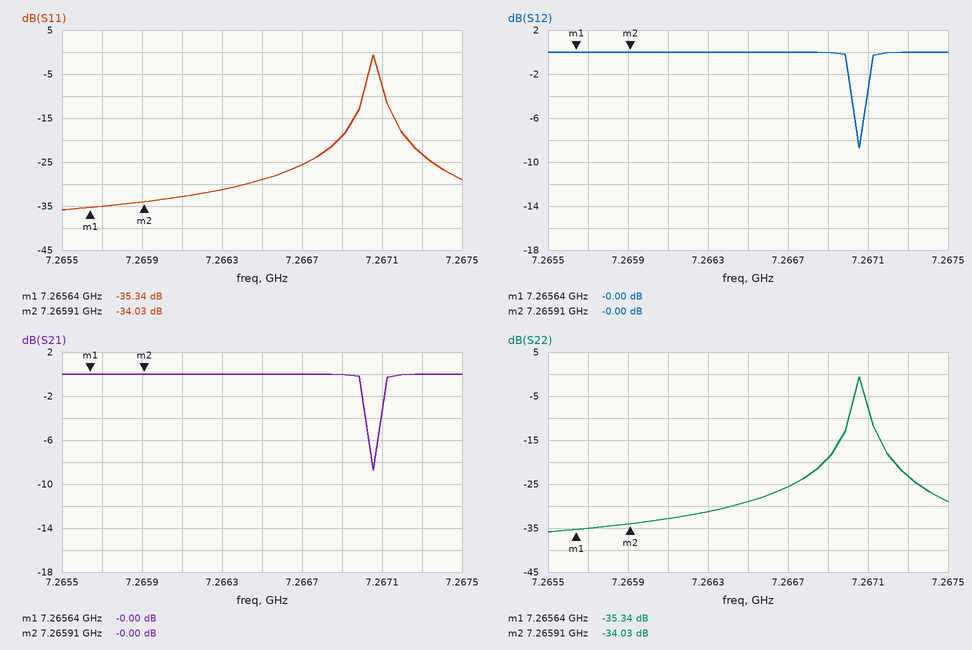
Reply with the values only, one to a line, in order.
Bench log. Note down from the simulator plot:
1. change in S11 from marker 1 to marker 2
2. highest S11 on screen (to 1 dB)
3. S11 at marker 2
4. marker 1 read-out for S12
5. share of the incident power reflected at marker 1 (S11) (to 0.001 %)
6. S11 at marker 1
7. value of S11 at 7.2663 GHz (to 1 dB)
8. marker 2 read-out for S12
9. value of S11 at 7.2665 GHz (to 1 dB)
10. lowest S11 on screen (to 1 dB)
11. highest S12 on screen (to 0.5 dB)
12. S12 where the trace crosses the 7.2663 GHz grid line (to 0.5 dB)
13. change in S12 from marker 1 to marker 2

1.31 dB
-1 dB
-34.03 dB
-0.00 dB
0.029 %
-35.34 dB
-31 dB
-0.00 dB
-29 dB
-36 dB
0.0 dB
0.0 dB
0.00 dB
